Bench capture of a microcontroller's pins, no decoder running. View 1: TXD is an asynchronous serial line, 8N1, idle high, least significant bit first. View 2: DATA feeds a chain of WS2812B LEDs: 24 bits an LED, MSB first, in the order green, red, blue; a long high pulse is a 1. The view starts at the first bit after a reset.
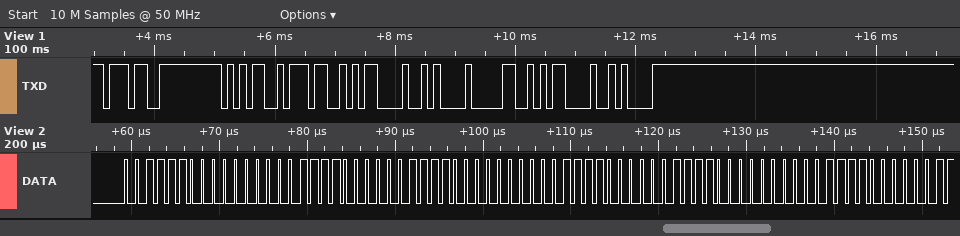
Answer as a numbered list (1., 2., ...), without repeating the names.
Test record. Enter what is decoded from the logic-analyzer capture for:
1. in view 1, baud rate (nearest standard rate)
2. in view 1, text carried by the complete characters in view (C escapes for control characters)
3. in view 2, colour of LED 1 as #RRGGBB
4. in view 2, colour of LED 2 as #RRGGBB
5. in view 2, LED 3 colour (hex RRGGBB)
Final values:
1. 9600 baud
2. "757\r\n0\r\n"
3. #003CF0
4. #003CF0
5. #003CF0
